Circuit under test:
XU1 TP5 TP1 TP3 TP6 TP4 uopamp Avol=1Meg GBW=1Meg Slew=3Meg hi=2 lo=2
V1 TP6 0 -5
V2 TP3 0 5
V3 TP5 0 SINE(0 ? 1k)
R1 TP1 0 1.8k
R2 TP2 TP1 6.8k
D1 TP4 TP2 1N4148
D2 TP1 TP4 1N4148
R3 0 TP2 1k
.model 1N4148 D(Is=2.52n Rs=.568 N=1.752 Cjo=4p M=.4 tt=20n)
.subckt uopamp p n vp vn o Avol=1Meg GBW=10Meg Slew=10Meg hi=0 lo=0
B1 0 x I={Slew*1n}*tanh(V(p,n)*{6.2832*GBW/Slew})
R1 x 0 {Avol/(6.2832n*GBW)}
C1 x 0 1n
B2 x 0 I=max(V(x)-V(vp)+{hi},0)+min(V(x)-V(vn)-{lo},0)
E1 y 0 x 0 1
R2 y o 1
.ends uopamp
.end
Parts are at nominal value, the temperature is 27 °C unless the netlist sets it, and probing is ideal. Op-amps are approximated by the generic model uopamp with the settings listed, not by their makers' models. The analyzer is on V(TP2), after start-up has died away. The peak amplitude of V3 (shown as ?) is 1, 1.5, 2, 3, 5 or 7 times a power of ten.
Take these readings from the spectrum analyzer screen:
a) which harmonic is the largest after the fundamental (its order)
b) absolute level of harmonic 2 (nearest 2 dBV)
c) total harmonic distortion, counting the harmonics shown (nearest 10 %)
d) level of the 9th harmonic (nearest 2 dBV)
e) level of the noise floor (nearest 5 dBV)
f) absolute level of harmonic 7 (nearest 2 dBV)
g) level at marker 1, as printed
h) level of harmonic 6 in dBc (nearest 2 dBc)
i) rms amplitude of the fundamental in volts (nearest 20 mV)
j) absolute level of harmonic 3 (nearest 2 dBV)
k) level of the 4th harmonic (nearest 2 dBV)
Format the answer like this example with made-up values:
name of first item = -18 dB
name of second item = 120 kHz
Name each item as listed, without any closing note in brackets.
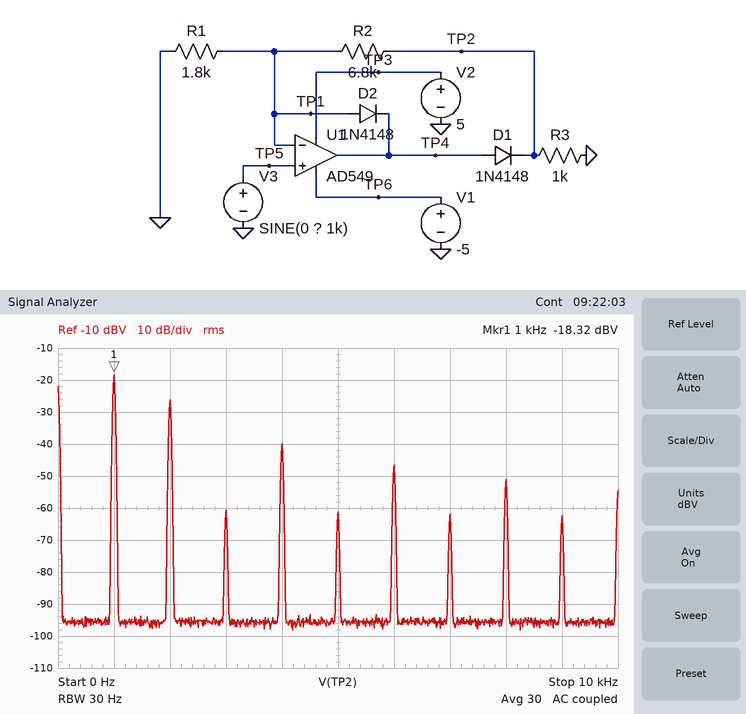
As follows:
which harmonic is the largest after the fundamental = 2
absolute level of harmonic 2 = -26 dBV
total harmonic distortion, counting the harmonics shown = 40 %
level of the 9th harmonic = -62 dBV
level of the noise floor = -95 dBV
absolute level of harmonic 7 = -62 dBV
level at marker 1, as printed = -18.32 dBV
level of harmonic 6 in dBc = -28 dBc
rms amplitude of the fundamental in volts = 120 mV
absolute level of harmonic 3 = -60 dBV
level of the 4th harmonic = -40 dBV
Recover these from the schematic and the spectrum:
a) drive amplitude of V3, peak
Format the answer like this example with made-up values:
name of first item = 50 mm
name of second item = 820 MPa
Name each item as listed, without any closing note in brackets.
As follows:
drive amplitude of V3, peak = 70 mV
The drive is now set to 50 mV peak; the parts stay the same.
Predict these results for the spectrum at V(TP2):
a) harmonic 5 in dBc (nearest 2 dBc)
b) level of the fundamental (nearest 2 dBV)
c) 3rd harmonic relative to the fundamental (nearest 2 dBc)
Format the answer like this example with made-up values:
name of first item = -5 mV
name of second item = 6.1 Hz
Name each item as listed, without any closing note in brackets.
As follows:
harmonic 5 in dBc = -40 dBc
level of the fundamental = -22 dBV
3rd harmonic relative to the fundamental = -40 dBc
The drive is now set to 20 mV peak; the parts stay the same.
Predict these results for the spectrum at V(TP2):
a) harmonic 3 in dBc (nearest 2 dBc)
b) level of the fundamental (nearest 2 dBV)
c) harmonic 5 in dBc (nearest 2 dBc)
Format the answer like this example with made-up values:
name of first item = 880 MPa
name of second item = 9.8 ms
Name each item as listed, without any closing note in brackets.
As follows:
harmonic 3 in dBc = -32 dBc
level of the fundamental = -30 dBV
harmonic 5 in dBc = -34 dBc
